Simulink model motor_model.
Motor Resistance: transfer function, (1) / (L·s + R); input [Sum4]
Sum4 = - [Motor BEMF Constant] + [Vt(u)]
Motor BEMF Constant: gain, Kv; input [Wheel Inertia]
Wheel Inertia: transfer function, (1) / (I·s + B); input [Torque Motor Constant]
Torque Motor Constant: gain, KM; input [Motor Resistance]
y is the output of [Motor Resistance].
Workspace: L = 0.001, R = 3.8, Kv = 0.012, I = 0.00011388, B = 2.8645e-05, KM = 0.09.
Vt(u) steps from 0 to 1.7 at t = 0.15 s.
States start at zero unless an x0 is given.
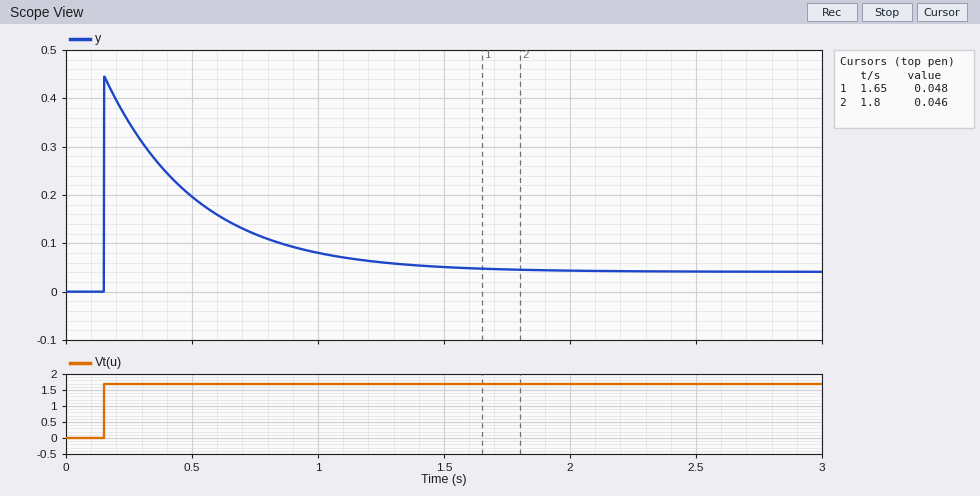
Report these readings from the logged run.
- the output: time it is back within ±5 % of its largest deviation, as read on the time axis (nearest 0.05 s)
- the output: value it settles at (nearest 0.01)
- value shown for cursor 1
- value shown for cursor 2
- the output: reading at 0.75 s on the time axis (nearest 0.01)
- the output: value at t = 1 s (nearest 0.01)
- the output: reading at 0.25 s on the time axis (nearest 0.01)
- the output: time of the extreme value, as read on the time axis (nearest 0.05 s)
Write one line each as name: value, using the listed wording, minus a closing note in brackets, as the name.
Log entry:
the output: time it is back within ±5 % of its largest deviation, as read on the time axis: 1.20 s
the output: value it settles at: 0.04
value shown for cursor 1: 0.048
value shown for cursor 2: 0.046
the output: reading at 0.75 s on the time axis: 0.12
the output: value at t = 1 s: 0.08
the output: reading at 0.25 s on the time axis: 0.35
the output: time of the extreme value, as read on the time axis: 0.15 s
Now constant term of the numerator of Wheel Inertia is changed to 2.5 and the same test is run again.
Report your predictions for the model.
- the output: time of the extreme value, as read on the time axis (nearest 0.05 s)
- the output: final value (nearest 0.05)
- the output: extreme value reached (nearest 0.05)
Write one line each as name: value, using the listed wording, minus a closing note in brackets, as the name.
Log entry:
the output: time of the extreme value, as read on the time axis: 0.15 s
the output: final value: 0.00
the output: extreme value reached: 0.45
